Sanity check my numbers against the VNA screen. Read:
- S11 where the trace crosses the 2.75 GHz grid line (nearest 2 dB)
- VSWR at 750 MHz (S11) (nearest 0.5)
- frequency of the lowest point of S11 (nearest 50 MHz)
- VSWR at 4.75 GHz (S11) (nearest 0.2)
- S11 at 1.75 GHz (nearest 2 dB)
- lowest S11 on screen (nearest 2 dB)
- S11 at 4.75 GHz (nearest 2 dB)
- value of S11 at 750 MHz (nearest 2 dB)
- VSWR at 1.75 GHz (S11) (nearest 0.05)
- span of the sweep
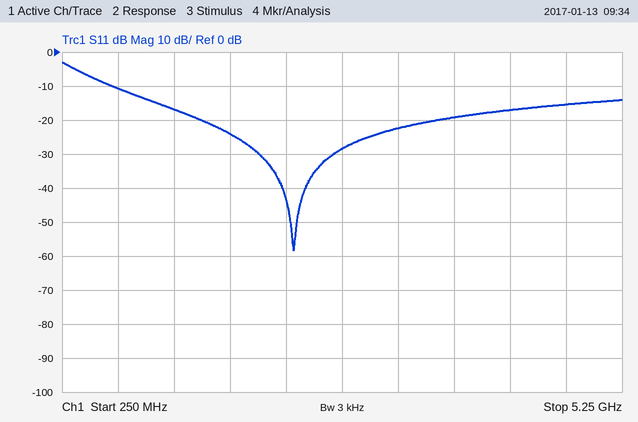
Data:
-28 dB
2.0
2.30 GHz
1.4
-24 dB
-58 dB
-16 dB
-10 dB
1.15
5 GHz
